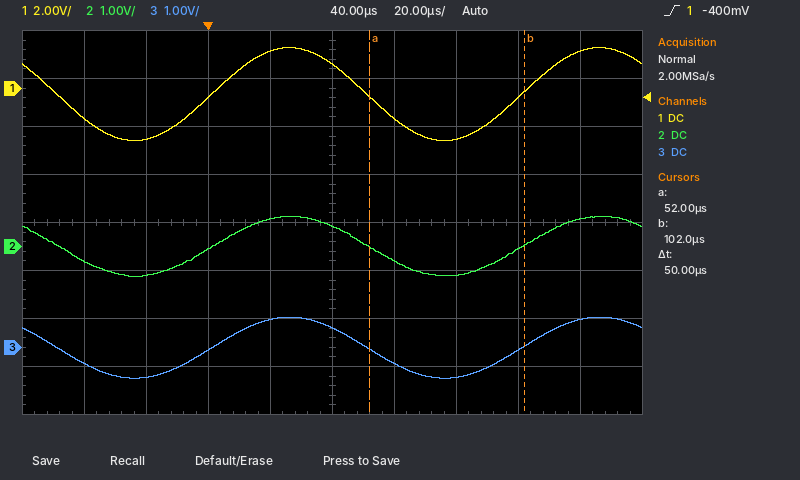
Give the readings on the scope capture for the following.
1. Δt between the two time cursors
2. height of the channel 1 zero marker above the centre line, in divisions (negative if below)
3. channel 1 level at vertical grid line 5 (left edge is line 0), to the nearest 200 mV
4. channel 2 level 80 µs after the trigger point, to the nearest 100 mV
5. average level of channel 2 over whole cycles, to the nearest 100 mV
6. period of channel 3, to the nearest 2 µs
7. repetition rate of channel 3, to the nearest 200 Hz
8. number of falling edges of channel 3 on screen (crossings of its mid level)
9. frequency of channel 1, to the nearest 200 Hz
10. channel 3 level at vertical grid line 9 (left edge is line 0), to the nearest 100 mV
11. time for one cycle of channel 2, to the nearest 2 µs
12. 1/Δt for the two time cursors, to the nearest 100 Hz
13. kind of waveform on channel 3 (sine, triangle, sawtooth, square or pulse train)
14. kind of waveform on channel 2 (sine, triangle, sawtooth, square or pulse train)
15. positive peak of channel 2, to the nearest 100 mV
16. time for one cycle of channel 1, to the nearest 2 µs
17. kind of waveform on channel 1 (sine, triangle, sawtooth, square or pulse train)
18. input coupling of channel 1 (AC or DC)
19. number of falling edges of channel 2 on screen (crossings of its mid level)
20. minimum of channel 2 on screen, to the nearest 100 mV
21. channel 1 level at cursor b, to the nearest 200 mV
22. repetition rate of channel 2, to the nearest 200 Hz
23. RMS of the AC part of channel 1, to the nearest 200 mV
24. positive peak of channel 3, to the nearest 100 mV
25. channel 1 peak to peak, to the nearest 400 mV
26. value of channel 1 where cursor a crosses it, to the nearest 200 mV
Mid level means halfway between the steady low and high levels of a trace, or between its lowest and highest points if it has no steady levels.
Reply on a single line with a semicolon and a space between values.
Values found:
50 µs; +2.8 div; 1.0 V; -600 mV; 0.0 V; 100 µs; 10.0 kHz; 2; 10.0 kHz; 600 mV; 100 µs; 20.0 kHz; sine; sine; 600 mV; 100 µs; sine; DC; 2; -600 mV; -200 mV; 10.0 kHz; 1.4 V; 600 mV; 4.0 V; -400 mV
